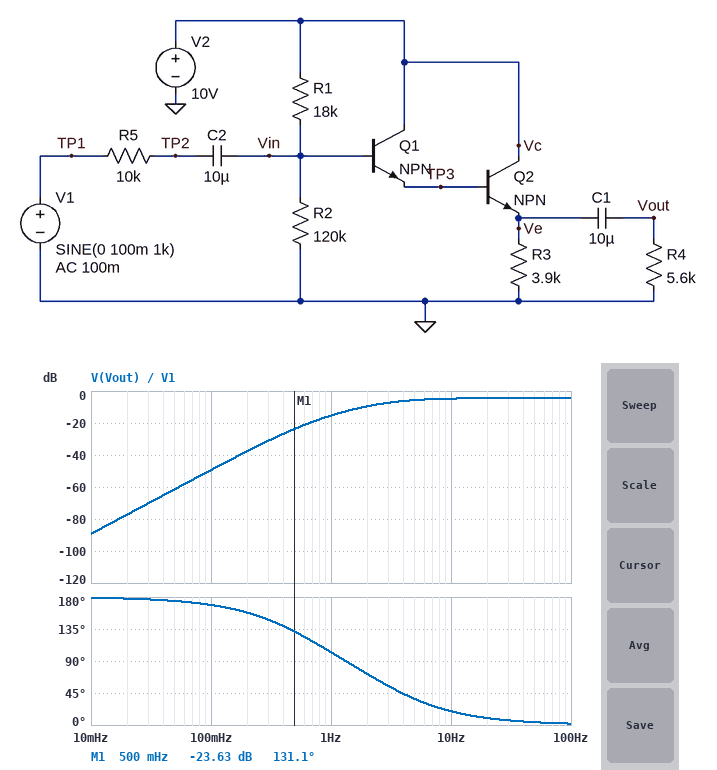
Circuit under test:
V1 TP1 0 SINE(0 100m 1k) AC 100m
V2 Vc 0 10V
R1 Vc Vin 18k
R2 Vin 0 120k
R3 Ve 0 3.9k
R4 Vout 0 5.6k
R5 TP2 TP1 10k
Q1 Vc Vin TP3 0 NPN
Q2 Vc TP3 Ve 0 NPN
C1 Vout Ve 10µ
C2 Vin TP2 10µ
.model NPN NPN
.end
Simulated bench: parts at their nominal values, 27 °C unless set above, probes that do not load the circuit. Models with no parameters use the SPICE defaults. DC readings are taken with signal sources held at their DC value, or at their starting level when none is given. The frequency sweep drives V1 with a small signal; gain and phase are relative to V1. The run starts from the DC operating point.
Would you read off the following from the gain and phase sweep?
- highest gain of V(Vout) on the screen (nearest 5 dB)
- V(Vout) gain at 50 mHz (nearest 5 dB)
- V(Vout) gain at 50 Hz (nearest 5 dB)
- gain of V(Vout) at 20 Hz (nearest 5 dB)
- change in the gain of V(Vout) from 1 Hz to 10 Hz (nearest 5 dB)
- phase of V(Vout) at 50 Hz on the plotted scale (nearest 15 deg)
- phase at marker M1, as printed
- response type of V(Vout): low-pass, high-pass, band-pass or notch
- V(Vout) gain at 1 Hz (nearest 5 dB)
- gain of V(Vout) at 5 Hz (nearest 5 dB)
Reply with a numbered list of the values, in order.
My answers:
1. -5 dB
2. -60 dB
3. -5 dB
4. -5 dB
5. 10 dB
6. 0 deg
7. 131.1 deg
8. high-pass
9. -15 dB
10. -5 dB
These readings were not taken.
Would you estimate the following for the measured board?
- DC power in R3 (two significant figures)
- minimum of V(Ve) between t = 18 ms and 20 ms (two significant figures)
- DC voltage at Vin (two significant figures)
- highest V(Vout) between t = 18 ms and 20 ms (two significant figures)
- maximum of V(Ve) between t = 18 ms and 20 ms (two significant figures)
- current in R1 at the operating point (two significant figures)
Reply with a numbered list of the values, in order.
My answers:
1. 13 mW
2. 7.2 V
3. 8.7 V
4. 60 mV
5. 7.3 V
6. 73 µA
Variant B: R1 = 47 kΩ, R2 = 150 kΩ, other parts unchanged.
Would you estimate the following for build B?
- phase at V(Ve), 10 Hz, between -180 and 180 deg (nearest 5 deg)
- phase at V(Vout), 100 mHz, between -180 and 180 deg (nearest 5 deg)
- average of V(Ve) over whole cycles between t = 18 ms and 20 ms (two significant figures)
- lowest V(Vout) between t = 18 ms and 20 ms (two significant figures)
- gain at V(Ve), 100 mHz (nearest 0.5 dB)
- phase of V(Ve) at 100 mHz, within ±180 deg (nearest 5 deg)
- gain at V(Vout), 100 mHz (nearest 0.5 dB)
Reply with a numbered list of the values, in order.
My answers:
1. 0 deg
2. 160 deg
3. 6.2 V
4. -77 mV
5. -13.5 dB
6. 75 deg
7. -42.5 dB
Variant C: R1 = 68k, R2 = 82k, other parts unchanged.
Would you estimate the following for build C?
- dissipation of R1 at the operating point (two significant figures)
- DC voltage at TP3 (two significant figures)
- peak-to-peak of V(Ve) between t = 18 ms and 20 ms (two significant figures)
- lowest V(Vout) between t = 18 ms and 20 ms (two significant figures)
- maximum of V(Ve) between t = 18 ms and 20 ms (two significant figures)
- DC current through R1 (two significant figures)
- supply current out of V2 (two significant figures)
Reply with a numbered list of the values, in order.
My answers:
1. 300 µW
2. 4.8 V
3. 150 mV
4. -77 mV
5. 4.1 V
6. 67 µA
7. 1.1 mA
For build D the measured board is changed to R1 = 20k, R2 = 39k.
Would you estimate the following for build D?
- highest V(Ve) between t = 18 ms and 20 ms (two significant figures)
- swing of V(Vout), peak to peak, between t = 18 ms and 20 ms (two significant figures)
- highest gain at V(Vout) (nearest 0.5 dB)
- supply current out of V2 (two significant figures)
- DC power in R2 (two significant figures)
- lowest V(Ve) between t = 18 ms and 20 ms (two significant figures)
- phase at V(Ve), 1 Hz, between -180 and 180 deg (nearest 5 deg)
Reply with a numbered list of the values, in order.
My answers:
1. 5.2 V
2. 110 mV
3. -5.0 dB
4. 1.5 mA
5. 1.1 mW
6. 5.1 V
7. 35 deg
